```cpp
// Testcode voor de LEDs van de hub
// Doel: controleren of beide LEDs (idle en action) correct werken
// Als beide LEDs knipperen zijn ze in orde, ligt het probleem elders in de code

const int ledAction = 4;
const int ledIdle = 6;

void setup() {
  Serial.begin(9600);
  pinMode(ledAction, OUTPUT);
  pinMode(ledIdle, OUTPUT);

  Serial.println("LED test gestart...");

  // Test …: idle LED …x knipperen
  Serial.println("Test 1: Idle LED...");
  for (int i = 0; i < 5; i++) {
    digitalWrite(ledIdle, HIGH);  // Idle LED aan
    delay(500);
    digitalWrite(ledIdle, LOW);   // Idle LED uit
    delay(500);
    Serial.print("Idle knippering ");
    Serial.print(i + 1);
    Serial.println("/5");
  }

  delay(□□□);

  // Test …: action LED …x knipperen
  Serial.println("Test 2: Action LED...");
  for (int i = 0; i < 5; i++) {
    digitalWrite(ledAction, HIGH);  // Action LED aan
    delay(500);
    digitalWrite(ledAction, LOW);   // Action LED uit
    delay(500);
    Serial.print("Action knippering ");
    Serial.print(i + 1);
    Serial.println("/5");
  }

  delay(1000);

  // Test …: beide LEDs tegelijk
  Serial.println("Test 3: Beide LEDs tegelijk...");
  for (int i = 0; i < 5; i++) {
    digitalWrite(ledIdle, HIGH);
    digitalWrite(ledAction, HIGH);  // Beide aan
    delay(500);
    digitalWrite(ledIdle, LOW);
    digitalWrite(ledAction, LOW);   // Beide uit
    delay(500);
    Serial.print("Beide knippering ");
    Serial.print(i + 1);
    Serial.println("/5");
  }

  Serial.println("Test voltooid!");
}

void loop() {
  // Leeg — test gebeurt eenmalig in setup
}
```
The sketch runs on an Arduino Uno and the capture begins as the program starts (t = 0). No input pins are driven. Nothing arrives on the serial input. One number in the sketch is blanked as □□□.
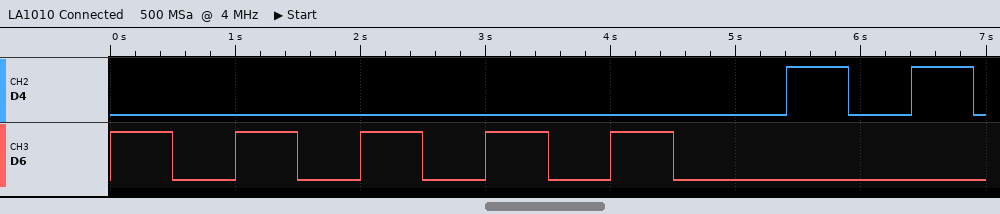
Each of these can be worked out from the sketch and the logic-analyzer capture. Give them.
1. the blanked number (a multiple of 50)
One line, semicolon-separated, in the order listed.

400
